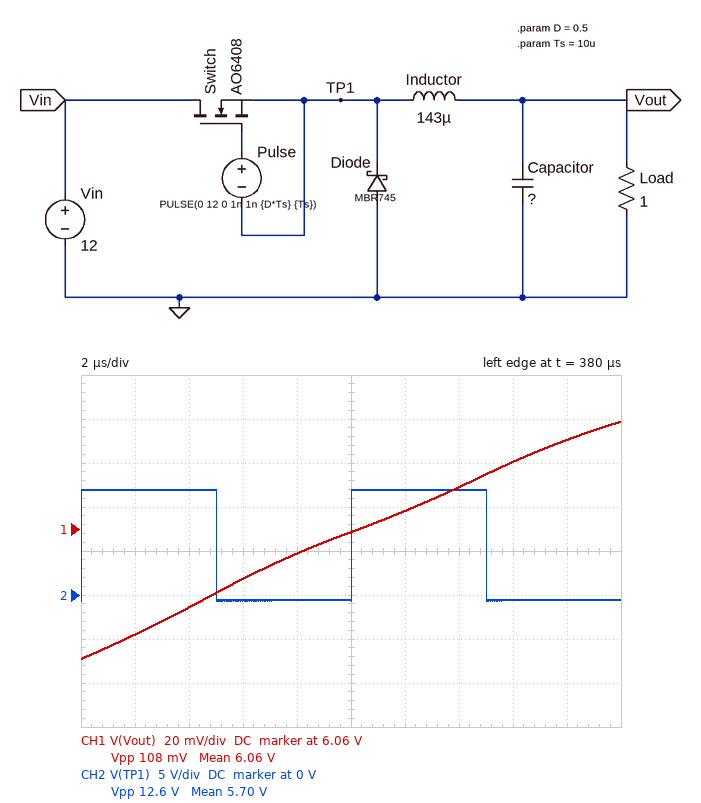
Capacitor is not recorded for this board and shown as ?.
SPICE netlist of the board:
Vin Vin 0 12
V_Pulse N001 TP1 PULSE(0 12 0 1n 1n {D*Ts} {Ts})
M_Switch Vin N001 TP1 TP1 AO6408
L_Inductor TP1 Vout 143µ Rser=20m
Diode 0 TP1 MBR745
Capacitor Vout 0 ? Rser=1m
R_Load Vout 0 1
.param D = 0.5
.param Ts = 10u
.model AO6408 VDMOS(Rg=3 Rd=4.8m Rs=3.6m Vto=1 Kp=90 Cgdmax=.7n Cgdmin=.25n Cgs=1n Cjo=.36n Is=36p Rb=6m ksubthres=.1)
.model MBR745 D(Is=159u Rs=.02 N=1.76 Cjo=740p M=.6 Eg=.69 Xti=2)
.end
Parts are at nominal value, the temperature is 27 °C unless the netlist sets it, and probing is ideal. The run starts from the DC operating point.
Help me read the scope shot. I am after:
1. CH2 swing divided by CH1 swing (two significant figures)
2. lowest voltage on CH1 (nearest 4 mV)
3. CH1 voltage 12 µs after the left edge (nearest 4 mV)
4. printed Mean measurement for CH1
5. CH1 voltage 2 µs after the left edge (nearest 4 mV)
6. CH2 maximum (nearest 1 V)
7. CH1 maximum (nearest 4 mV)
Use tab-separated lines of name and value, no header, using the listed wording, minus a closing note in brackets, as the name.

CH2 swing divided by CH1 swing	120
lowest voltage on CH1	6.000 V
CH1 voltage 12 µs after the left edge	6.068 V
printed Mean measurement for CH1	6.06 V
CH1 voltage 2 µs after the left edge	6.012 V
CH2 maximum	12 V
CH1 maximum	6.108 V
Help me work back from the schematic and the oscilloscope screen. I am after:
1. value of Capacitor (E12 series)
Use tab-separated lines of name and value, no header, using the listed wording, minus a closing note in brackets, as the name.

value of Capacitor	120 µF
